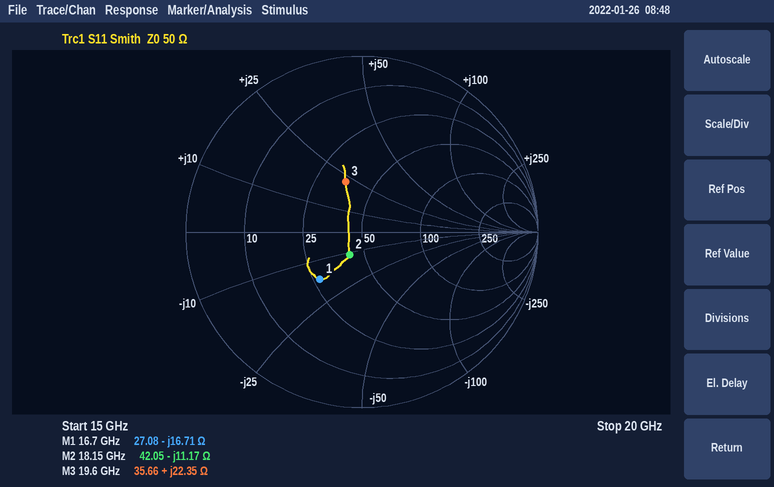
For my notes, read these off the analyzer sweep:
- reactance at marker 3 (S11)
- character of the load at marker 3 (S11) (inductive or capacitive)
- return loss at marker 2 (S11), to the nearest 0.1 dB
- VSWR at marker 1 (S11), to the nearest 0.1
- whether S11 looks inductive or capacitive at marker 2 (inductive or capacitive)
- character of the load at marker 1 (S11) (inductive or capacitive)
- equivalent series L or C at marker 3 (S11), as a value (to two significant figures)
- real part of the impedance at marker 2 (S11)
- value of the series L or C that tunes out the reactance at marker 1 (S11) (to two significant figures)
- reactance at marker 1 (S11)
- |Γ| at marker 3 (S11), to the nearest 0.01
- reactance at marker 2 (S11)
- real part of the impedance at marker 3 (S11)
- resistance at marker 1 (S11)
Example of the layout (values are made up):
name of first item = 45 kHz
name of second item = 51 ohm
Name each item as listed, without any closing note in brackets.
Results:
reactance at marker 3 = +22.35 Ω
character of the load at marker 3 (S11) = inductive
return loss at marker 2 (S11), to the nearest 0.1 dB = 16.6 dB
VSWR at marker 1 (S11), to the nearest 0.1 = 2.1
whether S11 looks inductive or capacitive at marker 2 = capacitive
character of the load at marker 1 (S11) = capacitive
equivalent series L or C at marker 3 (S11), as a value = 180 pH
real part of the impedance at marker 2 = 42.05 Ω
value of the series L or C that tunes out the reactance at marker 1 (S11) = 160 pH
reactance at marker 1 = -16.71 Ω
|Γ| at marker 3 (S11), to the nearest 0.01 = 0.30
reactance at marker 2 = -11.17 Ω
real part of the impedance at marker 3 = 35.66 Ω
resistance at marker 1 = 27.08 Ω
